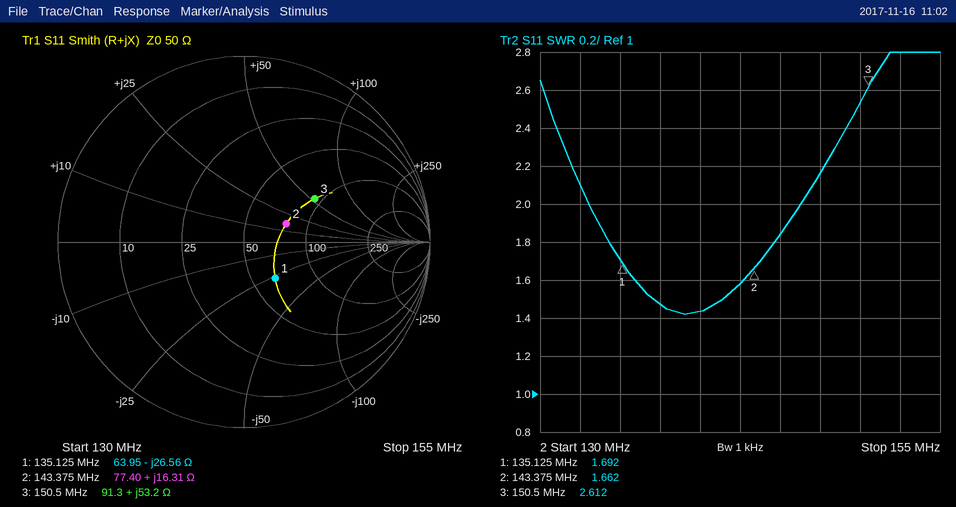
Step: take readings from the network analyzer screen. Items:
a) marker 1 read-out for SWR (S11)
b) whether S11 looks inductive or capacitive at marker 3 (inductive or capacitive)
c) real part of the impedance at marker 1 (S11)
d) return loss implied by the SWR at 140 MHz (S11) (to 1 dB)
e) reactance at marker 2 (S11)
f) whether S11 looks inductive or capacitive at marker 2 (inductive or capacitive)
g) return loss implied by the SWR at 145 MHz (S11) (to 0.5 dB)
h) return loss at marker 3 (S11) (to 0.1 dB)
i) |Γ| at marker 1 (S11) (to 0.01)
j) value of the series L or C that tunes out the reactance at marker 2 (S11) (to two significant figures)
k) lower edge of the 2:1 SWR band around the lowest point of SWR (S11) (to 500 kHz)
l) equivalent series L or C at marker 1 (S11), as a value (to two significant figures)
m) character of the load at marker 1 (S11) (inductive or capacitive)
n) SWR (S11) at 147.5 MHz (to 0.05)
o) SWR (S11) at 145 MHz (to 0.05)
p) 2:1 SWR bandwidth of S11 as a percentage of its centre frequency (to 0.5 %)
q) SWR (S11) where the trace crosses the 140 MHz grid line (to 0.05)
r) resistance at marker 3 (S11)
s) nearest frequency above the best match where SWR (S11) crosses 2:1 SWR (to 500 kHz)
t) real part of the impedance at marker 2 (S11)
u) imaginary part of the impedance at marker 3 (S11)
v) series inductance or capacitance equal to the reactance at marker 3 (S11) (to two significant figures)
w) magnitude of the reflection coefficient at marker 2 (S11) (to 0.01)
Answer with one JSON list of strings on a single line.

["1.692", "inductive", "63.95 Ω", "15 dB", "+16.31 Ω", "inductive", "10.5 dB", "7.0 dB", "0.26", "68 pF", "133.0 MHz", "44 pF", "capacitive", "2.15", "1.85", "9.5 %", "1.45", "91.3 Ω", "146.5 MHz", "77.40 Ω", "+53.2 Ω", "56 nH", "0.25"]
